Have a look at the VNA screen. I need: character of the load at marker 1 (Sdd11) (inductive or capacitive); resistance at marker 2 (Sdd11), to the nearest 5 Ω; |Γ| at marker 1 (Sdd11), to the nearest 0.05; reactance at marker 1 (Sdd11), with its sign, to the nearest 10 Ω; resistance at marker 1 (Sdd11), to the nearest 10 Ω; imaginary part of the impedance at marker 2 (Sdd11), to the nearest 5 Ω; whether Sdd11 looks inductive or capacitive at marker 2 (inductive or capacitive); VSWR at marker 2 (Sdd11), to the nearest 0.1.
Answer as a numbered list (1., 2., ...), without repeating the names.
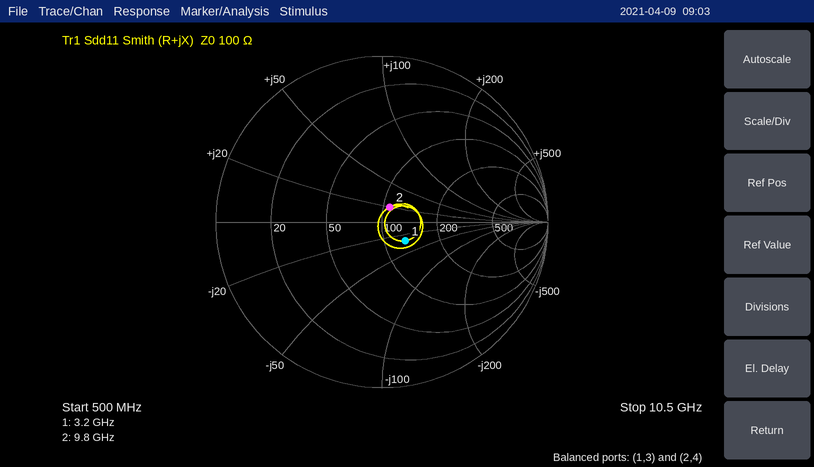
1. capacitive
2. 110 Ω
3. 0.20
4. -30 Ω
5. 130 Ω
6. +20 Ω
7. inductive
8. 1.2
